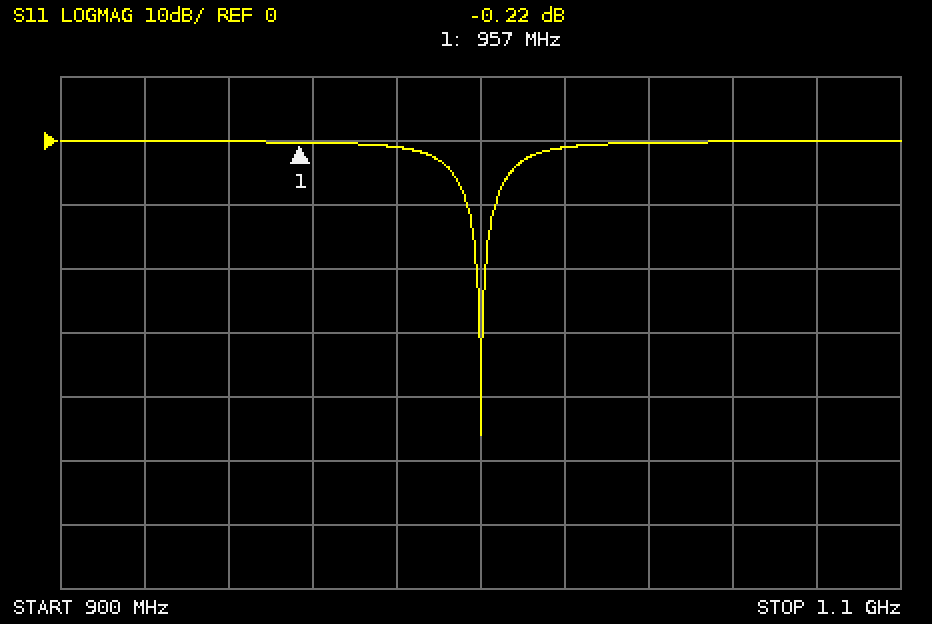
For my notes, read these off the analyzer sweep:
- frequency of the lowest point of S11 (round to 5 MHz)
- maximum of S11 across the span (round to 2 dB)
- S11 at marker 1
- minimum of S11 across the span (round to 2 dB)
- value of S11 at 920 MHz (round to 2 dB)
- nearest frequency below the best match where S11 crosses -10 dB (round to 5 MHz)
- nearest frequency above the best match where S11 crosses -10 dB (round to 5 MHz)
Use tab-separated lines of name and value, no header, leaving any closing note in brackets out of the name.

frequency of the lowest point of S11	1.000 GHz
maximum of S11 across the span	0 dB
S11 at marker 1	-0.22 dB
minimum of S11 across the span	-46 dB
value of S11 at 920 MHz	0 dB
nearest frequency below the best match where S11 crosses -10 dB	995 MHz
nearest frequency above the best match where S11 crosses -10 dB	1.005 GHz
